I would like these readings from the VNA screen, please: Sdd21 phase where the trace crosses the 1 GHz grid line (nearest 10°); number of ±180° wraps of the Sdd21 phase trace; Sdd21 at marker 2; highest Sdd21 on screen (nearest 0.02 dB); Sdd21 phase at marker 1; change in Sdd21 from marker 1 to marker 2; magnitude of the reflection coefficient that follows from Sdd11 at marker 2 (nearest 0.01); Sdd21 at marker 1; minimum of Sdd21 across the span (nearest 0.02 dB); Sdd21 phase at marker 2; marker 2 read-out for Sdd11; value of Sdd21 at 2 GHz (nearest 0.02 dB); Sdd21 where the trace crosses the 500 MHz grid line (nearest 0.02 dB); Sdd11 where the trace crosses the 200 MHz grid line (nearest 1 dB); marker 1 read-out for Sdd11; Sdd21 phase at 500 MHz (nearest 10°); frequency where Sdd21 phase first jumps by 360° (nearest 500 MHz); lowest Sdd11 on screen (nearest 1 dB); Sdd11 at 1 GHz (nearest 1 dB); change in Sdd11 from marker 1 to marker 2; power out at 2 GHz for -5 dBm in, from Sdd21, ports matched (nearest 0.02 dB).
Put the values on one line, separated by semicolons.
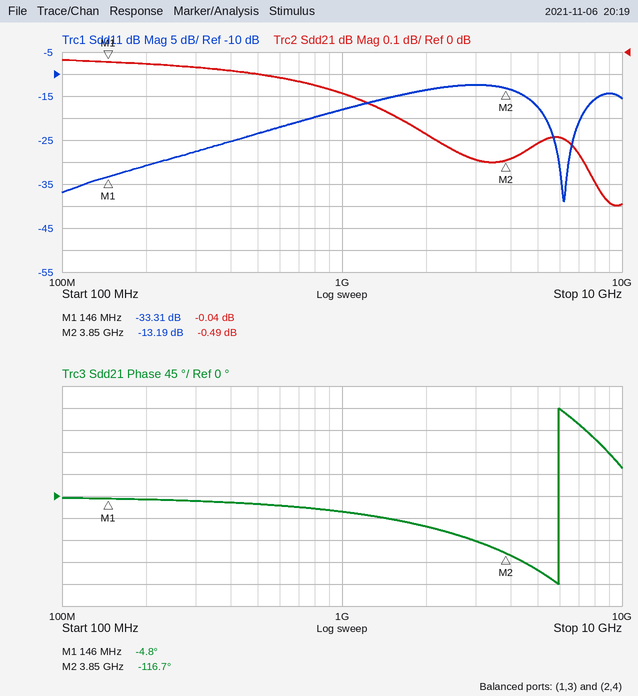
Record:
-30°; 1; -0.49 dB; -0.04 dB; -4.8°; -0.45 dB; 0.22; -0.04 dB; -0.70 dB; -116.7°; -13.19 dB; -0.38 dB; -0.10 dB; -31 dB; -33.31 dB; -20°; 6.0 GHz; -39 dB; -18 dB; 20.12 dB; -5.38 dBm
